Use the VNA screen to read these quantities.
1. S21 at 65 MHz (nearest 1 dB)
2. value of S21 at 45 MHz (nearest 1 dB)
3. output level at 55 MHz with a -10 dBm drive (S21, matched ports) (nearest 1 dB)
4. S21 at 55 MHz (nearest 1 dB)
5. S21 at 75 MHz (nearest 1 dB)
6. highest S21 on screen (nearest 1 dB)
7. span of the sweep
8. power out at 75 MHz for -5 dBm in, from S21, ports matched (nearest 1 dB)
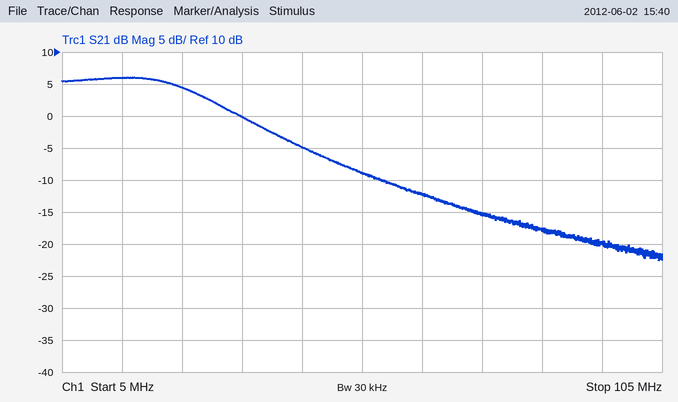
-12 dB
-5 dB
-19 dBm
-9 dB
-15 dB
6 dB
100 MHz
-20 dBm
